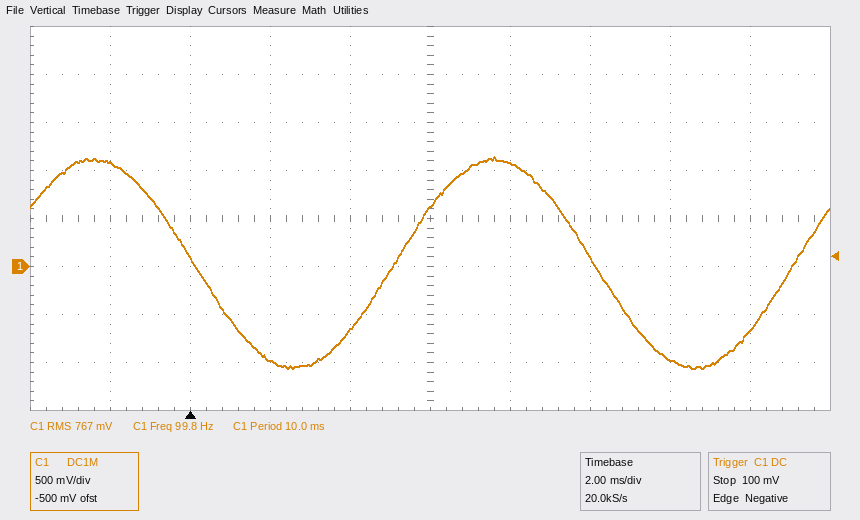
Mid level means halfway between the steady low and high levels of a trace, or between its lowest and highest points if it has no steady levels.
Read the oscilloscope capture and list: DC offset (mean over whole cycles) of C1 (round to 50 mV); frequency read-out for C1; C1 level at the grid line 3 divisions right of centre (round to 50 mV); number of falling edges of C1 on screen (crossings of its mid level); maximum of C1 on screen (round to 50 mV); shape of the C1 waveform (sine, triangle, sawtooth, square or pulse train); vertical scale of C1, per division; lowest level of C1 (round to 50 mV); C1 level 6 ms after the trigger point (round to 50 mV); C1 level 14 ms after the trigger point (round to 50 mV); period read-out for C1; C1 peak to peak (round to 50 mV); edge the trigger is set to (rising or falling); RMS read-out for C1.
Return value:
50 mV
99.8 Hz
-950 mV
2
1.15 V
sine
500 mV
-1.05 V
600 mV
-650 mV
10.0 ms
2.20 V
falling
767 mV
